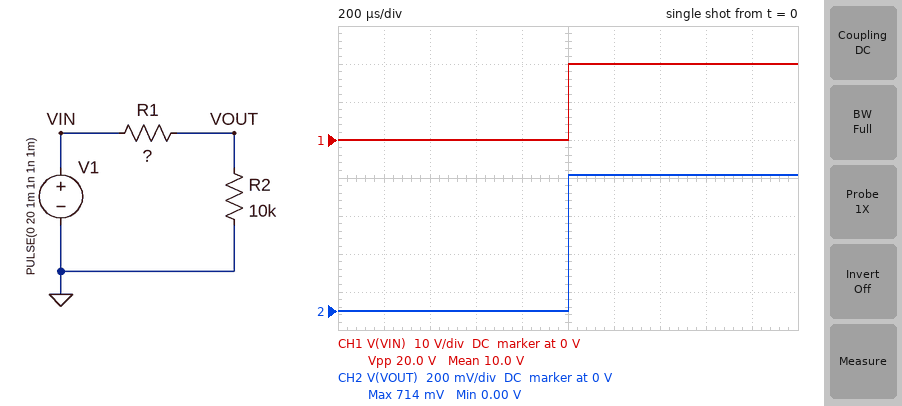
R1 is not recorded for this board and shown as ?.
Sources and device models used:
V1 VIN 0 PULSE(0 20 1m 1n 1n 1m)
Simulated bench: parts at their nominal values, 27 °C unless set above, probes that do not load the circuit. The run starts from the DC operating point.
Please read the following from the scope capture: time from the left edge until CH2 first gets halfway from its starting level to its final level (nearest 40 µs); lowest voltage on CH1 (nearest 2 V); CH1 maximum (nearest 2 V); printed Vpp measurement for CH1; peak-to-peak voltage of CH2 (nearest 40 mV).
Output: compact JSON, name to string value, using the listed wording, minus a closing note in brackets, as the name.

{"time from the left edge until CH2 first gets halfway from its starting level to its final level": "1.00 ms", "lowest voltage on CH1": "0 V", "CH1 maximum": "20 V", "printed Vpp measurement for CH1": "20.0 V", "peak-to-peak voltage of CH2": "720 mV"}
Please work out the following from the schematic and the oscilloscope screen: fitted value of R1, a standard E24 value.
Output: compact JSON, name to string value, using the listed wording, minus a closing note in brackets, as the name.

{"fitted value of R1, a standard E24 value": "270 kΩ"}
